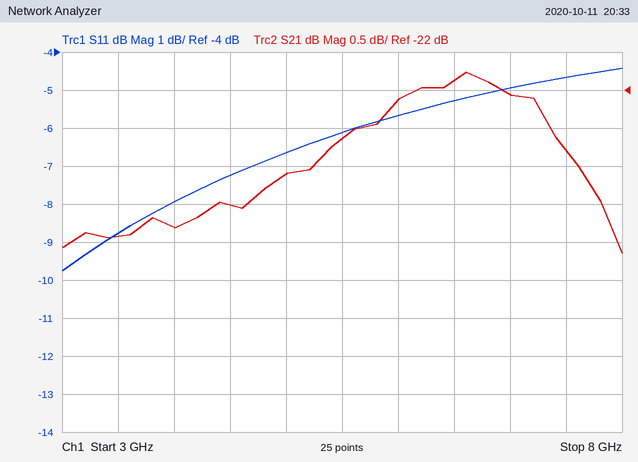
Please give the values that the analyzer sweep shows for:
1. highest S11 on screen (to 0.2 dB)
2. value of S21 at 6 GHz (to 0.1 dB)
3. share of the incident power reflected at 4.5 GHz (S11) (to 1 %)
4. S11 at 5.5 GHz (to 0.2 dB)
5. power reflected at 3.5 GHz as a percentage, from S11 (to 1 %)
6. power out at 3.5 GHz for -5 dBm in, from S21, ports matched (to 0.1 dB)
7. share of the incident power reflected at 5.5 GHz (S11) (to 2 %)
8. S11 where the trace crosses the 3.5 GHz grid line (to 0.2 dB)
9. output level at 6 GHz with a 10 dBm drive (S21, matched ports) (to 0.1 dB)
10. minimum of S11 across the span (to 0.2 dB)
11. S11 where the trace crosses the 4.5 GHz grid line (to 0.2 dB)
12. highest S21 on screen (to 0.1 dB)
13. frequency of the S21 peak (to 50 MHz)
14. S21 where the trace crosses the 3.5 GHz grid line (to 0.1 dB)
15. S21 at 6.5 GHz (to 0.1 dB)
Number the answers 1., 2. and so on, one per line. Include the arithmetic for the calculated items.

1. -4.4 dB
2. -22.1 dB
3. 10^(-7.2/10) ≈ 19 %
4. -6.2 dB
5. 10^(-8.8/10) ≈ 13 %
6. -5 dBm + (-23.9 dB) = -28.9 dBm
7. 10^(-6.2/10) ≈ 24 %
8. -8.8 dB
9. 10 dBm + (-22.1 dB) = -12.1 dBm
10. -9.8 dB
11. -7.2 dB
12. -21.8 dB
13. 6.60 GHz
14. -23.9 dB
15. -21.9 dB
